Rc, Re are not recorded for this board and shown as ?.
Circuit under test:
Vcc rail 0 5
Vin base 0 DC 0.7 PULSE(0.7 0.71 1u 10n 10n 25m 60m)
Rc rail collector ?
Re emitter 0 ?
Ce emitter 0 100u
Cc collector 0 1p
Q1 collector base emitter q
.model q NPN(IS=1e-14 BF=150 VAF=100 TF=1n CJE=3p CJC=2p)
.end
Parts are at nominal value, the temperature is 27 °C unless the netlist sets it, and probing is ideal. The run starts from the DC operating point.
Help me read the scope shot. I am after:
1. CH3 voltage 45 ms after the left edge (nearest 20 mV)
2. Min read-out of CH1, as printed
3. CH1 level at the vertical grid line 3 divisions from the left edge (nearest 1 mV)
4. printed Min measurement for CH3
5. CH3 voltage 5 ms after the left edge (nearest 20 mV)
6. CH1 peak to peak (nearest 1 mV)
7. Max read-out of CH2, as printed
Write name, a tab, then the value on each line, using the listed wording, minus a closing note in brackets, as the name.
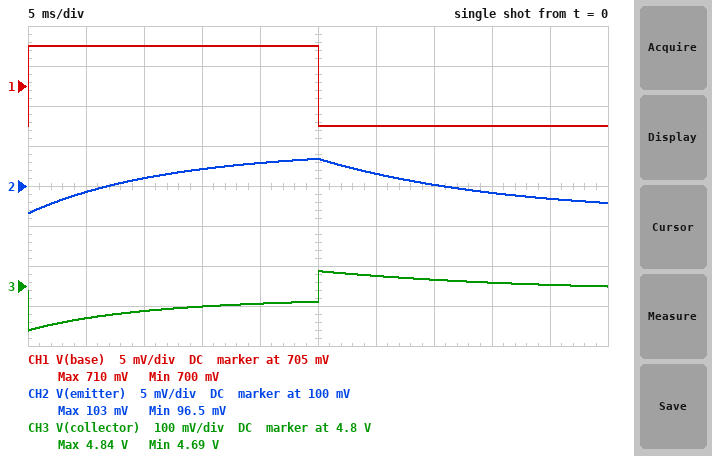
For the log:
CH3 voltage 45 ms after the left edge	4.80 V
Min read-out of CH1, as printed	700 mV
CH1 level at the vertical grid line 3 divisions from the left edge	710 mV
printed Min measurement for CH3	4.69 V
CH3 voltage 5 ms after the left edge	4.72 V
CH1 peak to peak	10 mV
Max read-out of CH2, as printed	103 mV
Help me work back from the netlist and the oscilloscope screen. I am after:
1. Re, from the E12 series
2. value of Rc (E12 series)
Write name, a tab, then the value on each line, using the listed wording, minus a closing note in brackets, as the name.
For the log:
Re, from the E12 series	680 Ω
value of Rc	1.5 kΩ
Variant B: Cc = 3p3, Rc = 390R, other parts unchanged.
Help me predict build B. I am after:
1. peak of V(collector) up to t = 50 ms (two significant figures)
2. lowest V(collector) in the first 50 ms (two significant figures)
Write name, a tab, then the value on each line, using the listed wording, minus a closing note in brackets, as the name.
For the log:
peak of V(collector) up to t = 50 ms	5.0 V
lowest V(collector) in the first 50 ms	4.9 V
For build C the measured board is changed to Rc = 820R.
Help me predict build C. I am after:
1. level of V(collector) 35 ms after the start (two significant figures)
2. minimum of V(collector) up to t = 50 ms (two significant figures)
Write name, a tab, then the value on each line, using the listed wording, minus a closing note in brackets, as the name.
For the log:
level of V(collector) 35 ms after the start	4.9 V
minimum of V(collector) up to t = 50 ms	4.8 V
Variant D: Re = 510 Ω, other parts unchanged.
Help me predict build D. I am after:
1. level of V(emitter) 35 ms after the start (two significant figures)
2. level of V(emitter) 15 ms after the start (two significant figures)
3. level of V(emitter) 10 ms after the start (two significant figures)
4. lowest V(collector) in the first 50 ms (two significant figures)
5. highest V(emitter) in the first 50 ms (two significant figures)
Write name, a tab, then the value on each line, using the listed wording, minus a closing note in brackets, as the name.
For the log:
level of V(emitter) 35 ms after the start	94 mV
level of V(emitter) 15 ms after the start	97 mV
level of V(emitter) 10 ms after the start	96 mV
lowest V(collector) in the first 50 ms	4.6 V
highest V(emitter) in the first 50 ms	98 mV
